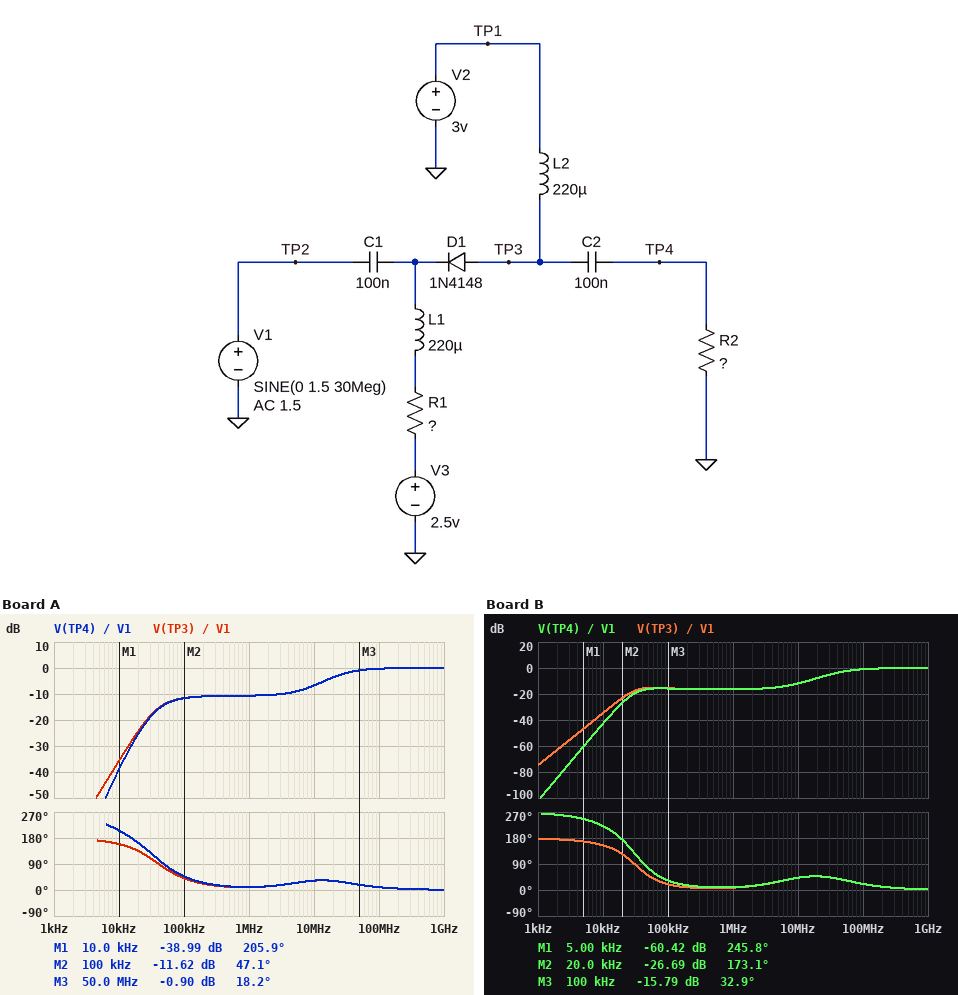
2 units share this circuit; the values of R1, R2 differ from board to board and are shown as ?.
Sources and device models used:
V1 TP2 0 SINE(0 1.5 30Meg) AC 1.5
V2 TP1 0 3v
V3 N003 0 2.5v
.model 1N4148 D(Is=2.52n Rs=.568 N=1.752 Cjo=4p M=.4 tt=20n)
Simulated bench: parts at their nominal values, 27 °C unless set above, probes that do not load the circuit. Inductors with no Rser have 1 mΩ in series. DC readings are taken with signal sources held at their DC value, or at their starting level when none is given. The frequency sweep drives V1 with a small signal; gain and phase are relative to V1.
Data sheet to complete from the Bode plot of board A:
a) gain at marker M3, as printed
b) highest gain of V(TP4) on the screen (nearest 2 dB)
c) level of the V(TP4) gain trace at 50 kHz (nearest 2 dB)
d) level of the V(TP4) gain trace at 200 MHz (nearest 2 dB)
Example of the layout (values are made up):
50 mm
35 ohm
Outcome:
-0.90 dB
0 dB
-14 dB
0 dB
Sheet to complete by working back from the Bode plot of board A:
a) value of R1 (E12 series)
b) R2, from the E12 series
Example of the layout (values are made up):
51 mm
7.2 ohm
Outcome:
82 Ω
150 Ω
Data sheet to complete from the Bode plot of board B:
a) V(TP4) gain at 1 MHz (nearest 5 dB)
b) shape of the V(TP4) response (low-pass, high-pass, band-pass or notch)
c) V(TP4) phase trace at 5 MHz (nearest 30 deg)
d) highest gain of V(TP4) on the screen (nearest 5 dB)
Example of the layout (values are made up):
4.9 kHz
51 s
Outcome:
-15 dB
high-pass
30 deg
0 dB
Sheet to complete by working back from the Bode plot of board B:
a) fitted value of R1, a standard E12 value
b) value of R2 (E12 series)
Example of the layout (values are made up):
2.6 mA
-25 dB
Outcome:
100 Ω
68 Ω
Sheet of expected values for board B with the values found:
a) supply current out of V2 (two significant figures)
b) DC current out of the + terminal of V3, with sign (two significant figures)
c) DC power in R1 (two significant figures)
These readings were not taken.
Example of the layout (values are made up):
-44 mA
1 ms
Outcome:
120 µA
-120 µA
1.4 µW
